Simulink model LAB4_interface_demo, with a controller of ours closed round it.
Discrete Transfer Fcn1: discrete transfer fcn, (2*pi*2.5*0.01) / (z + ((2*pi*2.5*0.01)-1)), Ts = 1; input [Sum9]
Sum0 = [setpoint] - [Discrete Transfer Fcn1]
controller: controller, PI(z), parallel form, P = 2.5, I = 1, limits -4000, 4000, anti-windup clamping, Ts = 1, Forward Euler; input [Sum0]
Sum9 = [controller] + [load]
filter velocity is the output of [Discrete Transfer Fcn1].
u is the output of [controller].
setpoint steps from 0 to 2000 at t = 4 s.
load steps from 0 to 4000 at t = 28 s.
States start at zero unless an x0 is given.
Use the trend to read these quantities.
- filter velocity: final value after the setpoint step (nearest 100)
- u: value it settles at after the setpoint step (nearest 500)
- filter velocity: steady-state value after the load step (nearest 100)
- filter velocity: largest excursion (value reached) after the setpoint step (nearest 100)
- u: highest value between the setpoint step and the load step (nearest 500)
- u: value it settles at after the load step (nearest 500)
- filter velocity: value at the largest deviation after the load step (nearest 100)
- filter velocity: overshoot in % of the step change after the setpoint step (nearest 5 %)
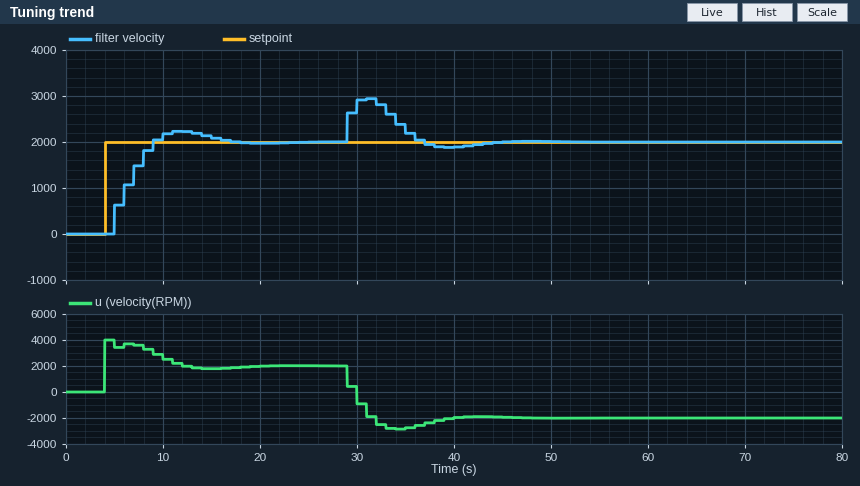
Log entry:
2000
2000
2000
2200
4000
-2000
2900
10 %
